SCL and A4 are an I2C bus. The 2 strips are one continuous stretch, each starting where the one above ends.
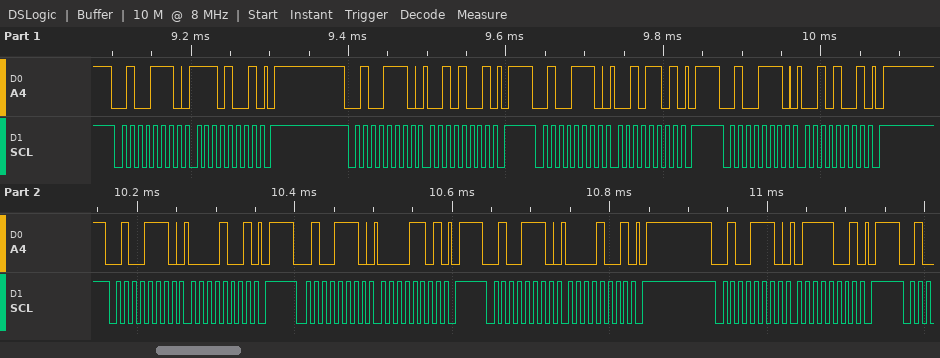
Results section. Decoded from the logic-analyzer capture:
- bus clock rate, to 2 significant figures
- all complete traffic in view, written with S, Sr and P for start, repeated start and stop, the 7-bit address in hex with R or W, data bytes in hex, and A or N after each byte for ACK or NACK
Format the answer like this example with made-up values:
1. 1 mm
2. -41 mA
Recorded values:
1. 100 kHz
2. S 27W A E9 A P S 27W A 29 A P S 27W A 2D A P S 27W A 29 A P S 27W A 09 A P S 27W A 0D A P S 27W A 09 A P S 27W A 79 A P
